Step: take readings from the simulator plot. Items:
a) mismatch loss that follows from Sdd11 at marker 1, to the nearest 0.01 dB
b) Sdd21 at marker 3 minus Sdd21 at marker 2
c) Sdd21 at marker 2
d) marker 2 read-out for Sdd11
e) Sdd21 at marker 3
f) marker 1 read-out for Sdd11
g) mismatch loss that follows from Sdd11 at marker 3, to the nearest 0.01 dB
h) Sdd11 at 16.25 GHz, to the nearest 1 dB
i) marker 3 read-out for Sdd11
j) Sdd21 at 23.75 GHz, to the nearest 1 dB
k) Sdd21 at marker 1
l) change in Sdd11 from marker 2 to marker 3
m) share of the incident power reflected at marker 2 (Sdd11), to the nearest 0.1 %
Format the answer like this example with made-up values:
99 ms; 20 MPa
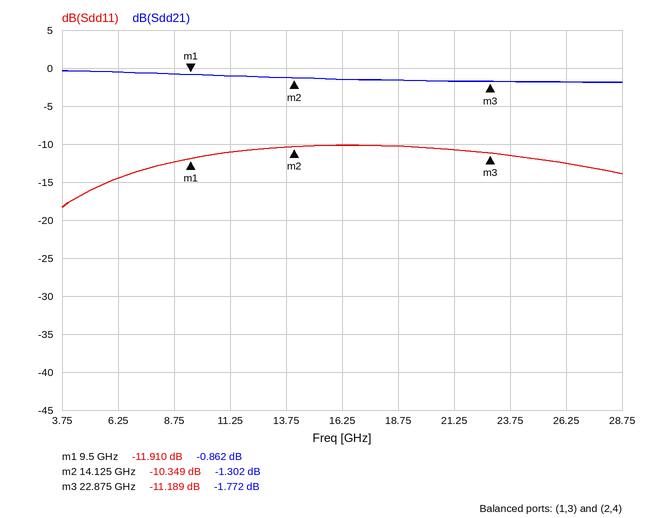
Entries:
0.29 dB; -0.470 dB; -1.302 dB; -10.349 dB; -1.772 dB; -11.910 dB; 0.34 dB; -10 dB; -11.189 dB; -2 dB; -0.862 dB; -0.840 dB; 9.2 %
